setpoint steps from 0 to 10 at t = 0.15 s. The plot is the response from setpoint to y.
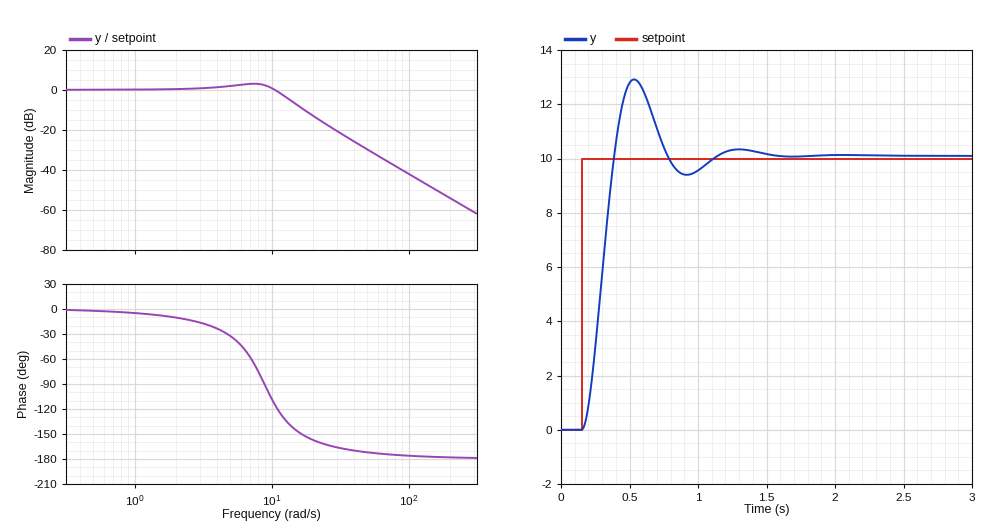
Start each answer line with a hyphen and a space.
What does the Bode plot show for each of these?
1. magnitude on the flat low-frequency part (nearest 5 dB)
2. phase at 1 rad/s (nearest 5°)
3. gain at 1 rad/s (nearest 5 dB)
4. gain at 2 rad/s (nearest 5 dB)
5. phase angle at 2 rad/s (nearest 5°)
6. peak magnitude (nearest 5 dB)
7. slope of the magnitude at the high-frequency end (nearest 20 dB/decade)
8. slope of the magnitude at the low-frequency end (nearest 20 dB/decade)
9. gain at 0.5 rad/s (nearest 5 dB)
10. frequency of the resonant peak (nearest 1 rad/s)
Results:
- 0 dB
- -5°
- 0 dB
- 0 dB
- -10°
- 5 dB
- -40 dB/decade
- 0 dB/decade
- 0 dB
- 7 rad/s
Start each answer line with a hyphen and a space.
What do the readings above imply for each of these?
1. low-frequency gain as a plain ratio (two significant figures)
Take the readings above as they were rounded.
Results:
- 1.0
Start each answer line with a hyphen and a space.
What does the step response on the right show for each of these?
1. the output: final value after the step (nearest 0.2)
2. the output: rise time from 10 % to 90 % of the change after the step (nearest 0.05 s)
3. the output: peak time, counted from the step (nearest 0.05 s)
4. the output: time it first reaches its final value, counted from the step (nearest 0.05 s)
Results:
- 10.0
- 0.15 s
- 0.40 s
- 0.25 s
